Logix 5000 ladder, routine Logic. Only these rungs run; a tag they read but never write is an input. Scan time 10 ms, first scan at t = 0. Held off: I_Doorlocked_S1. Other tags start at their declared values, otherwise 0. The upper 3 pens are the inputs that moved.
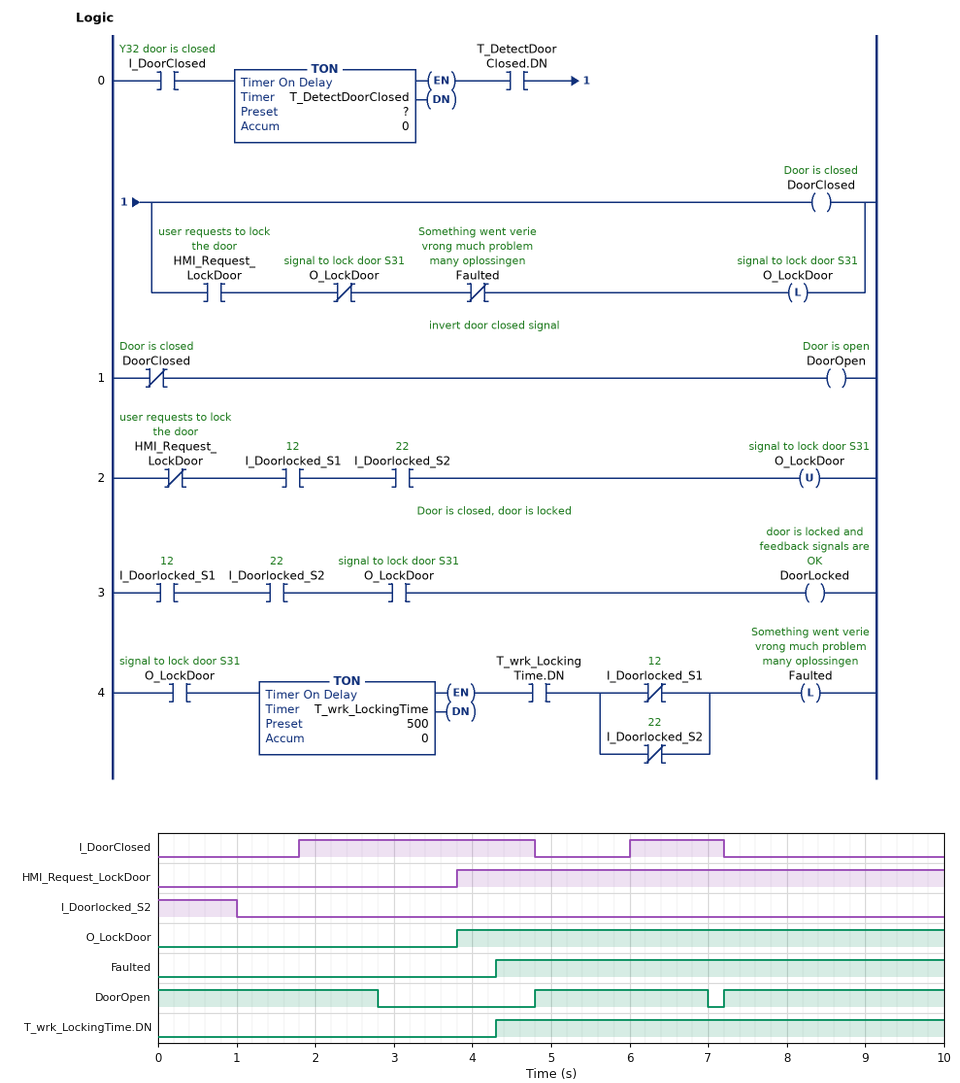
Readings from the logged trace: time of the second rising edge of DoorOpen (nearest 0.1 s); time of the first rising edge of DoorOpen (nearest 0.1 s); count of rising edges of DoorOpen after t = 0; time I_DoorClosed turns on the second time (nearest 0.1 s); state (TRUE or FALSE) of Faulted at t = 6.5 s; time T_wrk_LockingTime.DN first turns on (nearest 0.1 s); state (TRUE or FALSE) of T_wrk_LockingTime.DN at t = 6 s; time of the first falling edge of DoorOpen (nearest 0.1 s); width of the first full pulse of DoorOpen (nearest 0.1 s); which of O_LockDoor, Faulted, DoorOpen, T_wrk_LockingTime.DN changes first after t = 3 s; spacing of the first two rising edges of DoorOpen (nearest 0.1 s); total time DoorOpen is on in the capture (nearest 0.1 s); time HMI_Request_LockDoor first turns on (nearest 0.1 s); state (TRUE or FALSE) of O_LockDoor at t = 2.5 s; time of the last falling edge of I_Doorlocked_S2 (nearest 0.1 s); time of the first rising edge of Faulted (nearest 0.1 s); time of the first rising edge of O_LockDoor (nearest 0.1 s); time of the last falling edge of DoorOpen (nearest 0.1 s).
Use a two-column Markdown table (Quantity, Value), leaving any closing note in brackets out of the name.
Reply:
| Quantity | Value |
|---|---|
| time of the second rising edge of DoorOpen | 7.2 s |
| time of the first rising edge of DoorOpen | 4.8 s |
| count of rising edges of DoorOpen after t = 0 | 2 |
| time I_DoorClosed turns on the second time | 6.0 s |
| state (TRUE or FALSE) of Faulted at t = 6.5 s | TRUE |
| time T_wrk_LockingTime.DN first turns on | 4.3 s |
| state (TRUE or FALSE) of T_wrk_LockingTime.DN at t = 6 s | TRUE |
| time of the first falling edge of DoorOpen | 2.8 s |
| width of the first full pulse of DoorOpen | 2.2 s |
| which of O_LockDoor, Faulted, DoorOpen, T_wrk_LockingTime.DN changes first after t = 3 s | O_LockDoor |
| spacing of the first two rising edges of DoorOpen | 2.4 s |
| total time DoorOpen is on in the capture | 7.8 s |
| time HMI_Request_LockDoor first turns on | 3.8 s |
| state (TRUE or FALSE) of O_LockDoor at t = 2.5 s | FALSE |
| time of the last falling edge of I_Doorlocked_S2 | 1.0 s |
| time of the first rising edge of Faulted | 4.3 s |
| time of the first rising edge of O_LockDoor | 3.8 s |
| time of the last falling edge of DoorOpen | 7.0 s |
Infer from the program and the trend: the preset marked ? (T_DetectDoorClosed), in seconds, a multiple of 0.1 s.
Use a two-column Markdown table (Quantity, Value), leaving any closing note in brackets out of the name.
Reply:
| Quantity | Value |
|---|---|
| the preset marked ? (T_DetectDoorClosed), in seconds, a multiple of 0.1 s | 1.0 s |
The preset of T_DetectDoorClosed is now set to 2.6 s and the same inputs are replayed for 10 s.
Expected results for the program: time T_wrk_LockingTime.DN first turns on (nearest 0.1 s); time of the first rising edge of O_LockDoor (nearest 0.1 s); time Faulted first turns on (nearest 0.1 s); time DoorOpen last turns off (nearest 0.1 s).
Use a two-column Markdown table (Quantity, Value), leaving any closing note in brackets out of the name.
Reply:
| Quantity | Value |
|---|---|
| time T_wrk_LockingTime.DN first turns on | 4.9 s |
| time of the first rising edge of O_LockDoor | 4.4 s |
| time Faulted first turns on | 4.9 s |
| time DoorOpen last turns off | 4.4 s |
